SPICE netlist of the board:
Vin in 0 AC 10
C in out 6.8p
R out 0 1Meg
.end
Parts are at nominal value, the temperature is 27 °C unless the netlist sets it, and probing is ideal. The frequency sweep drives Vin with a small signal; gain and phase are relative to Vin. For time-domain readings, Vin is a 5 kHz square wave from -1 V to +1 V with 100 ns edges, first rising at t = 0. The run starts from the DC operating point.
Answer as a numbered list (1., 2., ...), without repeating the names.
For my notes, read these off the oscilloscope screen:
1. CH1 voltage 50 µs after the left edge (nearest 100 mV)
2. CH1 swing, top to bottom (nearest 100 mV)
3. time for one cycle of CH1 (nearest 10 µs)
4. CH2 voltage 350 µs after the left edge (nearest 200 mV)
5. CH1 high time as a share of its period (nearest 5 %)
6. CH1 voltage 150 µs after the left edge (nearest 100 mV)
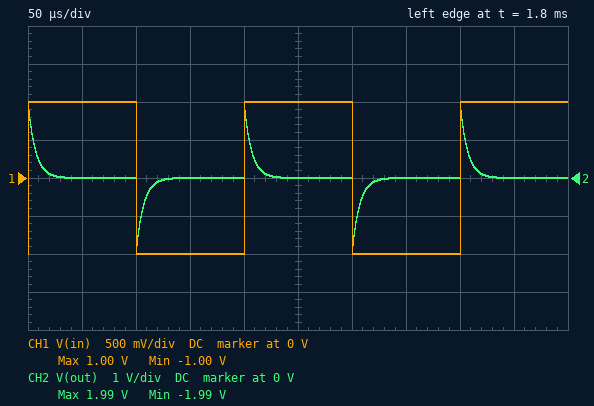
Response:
1. 1.0 V
2. 2.0 V
3. 200 µs
4. 0 V
5. 50 %
6. -1.0 V
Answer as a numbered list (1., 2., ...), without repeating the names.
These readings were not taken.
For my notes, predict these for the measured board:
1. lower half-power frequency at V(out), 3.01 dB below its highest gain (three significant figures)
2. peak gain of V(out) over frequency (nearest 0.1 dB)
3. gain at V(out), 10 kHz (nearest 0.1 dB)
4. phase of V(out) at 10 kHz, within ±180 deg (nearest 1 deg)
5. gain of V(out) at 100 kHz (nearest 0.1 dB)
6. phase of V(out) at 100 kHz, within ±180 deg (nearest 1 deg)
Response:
1. 23.4 kHz
2. 0 dB
3. -8.1 dB
4. 67 deg
5. -0.2 dB
6. 13 deg
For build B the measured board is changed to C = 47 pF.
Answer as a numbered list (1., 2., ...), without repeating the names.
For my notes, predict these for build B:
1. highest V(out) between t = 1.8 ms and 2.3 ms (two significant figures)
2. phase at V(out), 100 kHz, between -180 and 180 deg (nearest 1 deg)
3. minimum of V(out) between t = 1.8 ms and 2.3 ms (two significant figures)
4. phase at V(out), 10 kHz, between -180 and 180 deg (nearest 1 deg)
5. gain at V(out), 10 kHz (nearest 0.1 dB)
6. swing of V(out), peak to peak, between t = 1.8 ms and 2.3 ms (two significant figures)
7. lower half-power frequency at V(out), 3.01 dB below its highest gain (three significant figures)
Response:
1. 1.8 V
2. 2 deg
3. -1.8 V
4. 19 deg
5. -0.5 dB
6. 3.6 V
7. 3.39 kHz
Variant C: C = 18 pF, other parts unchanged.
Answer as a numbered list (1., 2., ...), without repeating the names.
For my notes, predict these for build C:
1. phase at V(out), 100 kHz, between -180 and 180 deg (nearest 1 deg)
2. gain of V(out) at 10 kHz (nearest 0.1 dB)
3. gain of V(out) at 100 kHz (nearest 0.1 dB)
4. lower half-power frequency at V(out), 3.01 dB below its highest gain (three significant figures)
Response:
1. 5 deg
2. -2.5 dB
3. 0 dB
4. 8.84 kHz
